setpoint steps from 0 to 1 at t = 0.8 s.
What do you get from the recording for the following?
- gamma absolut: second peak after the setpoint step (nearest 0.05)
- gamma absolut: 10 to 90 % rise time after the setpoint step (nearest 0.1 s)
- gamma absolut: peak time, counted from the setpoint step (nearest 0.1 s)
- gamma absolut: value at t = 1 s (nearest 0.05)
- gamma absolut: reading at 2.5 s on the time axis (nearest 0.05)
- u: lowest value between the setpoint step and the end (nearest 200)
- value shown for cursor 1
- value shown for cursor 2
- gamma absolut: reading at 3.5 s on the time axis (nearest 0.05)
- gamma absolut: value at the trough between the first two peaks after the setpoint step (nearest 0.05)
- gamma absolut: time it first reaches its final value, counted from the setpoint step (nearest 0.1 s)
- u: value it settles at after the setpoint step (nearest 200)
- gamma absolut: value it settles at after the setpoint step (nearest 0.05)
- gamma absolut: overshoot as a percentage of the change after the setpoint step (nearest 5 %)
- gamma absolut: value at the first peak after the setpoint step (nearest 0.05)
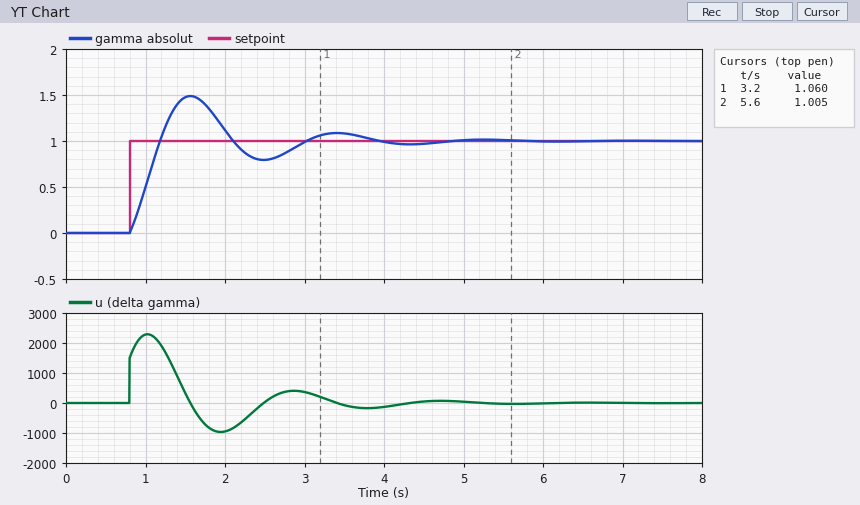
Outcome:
1.10
0.3 s
0.8 s
0.50
0.80
-1000
1.060
1.005
1.10
0.80
0.4 s
0
1.00
50 %
1.50
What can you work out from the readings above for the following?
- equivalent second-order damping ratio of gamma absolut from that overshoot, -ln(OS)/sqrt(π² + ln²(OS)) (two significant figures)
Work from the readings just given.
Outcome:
0.22
